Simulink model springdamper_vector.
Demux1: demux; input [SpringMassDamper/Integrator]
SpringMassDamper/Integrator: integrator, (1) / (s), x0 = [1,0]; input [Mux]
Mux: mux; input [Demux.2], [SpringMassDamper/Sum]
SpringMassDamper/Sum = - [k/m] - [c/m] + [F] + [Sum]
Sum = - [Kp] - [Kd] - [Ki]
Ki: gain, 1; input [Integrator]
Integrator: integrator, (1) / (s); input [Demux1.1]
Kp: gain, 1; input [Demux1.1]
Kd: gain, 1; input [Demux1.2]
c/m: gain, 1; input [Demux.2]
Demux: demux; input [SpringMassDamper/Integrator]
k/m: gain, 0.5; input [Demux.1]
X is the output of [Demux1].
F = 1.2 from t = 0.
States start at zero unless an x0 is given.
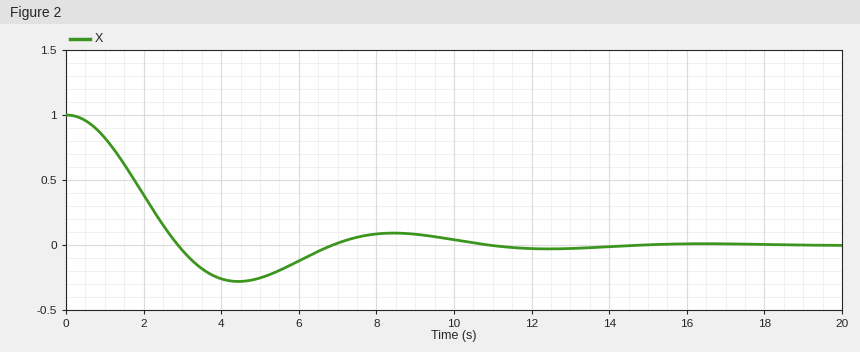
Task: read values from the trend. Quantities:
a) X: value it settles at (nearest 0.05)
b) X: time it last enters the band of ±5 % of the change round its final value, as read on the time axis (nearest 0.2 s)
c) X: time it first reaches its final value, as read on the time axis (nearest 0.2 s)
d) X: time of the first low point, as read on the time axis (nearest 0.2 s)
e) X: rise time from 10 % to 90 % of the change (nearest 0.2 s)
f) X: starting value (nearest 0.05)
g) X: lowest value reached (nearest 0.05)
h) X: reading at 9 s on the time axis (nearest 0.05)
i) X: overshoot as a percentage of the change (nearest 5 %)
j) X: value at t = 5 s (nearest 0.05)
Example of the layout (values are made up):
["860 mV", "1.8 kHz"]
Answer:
["0.00", "9.8 s", "2.8 s", "4.4 s", "1.8 s", "1.00", "-0.30", "0.10", "30 %", "-0.25"]
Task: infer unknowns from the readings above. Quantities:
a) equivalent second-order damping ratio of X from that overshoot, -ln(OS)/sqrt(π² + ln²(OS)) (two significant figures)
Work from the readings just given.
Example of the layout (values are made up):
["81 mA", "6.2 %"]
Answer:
["0.36"]
